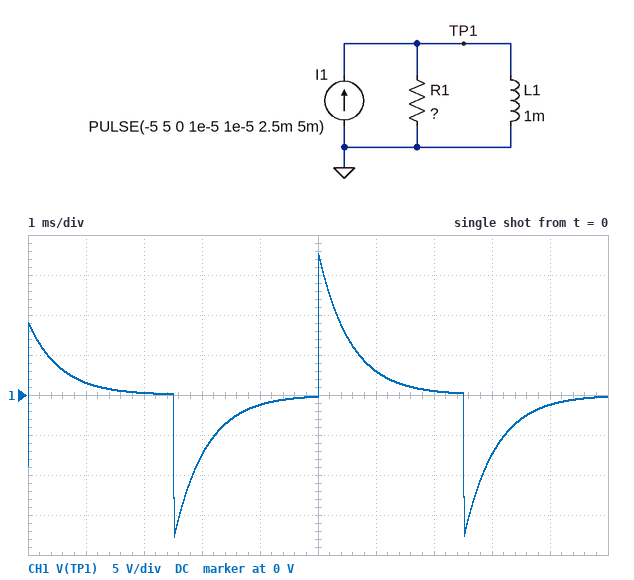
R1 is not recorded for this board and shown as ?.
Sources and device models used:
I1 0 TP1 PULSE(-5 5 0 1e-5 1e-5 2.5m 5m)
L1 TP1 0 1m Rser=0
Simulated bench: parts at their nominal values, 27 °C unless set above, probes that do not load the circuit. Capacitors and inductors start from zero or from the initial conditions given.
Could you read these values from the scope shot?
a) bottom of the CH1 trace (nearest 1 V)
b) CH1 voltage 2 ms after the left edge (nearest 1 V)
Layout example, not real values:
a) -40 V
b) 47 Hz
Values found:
a) -18 V
b) 0 V
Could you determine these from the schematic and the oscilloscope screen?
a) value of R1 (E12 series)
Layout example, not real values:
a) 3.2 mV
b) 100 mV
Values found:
a) 1.8 Ω
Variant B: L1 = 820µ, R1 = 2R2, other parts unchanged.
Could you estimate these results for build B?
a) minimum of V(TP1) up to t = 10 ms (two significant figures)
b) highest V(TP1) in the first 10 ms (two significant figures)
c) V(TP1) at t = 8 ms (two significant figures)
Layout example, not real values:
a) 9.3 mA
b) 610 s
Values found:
a) -22 V
b) 22 V
c) -6.0 V
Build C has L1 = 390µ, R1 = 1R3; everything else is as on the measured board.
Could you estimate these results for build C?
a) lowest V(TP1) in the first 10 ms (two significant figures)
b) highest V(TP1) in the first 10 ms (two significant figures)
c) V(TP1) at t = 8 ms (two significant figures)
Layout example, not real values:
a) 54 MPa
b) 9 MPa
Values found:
a) -13 V
b) 13 V
c) -2.6 V
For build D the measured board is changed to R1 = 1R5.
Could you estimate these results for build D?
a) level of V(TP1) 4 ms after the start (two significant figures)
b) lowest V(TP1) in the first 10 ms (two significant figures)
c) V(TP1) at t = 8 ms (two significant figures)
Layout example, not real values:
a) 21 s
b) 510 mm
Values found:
a) -1.6 V
b) -15 V
c) -7.1 V
